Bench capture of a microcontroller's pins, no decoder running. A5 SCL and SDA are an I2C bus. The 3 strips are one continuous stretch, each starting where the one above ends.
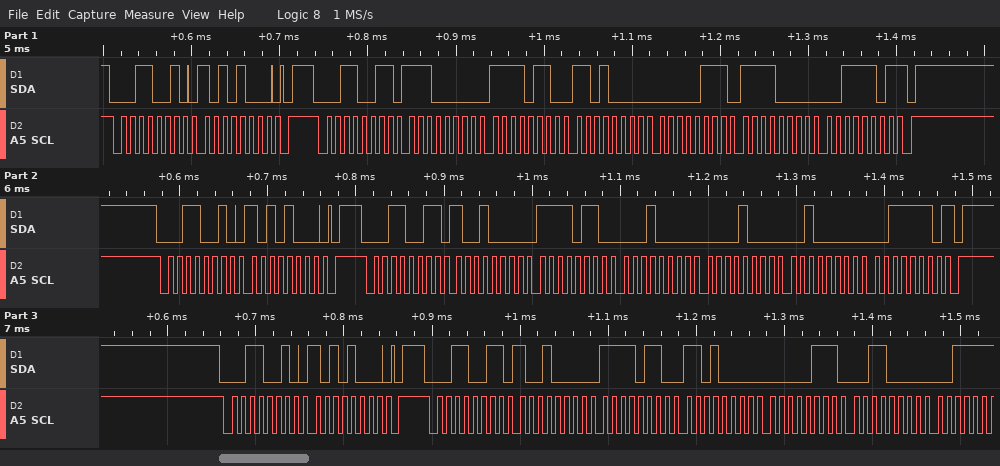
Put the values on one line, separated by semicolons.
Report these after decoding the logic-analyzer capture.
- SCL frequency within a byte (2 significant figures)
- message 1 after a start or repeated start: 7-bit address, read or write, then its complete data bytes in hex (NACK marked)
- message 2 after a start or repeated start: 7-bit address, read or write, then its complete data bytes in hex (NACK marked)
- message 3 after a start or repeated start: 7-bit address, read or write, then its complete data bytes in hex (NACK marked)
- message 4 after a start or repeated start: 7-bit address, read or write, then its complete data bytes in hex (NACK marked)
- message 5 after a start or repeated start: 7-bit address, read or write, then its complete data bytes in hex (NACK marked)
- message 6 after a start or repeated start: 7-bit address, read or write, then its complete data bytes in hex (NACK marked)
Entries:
100 kHz; 0x19 write: A8; 0x19 read: E0 F6 D0 07 F0 3D NACK; 0x19 write: A8; 0x19 read: 90 F6 10 08 20 3E NACK; 0x19 write: A8; 0x19 read: 90 F6 D0 07 30
